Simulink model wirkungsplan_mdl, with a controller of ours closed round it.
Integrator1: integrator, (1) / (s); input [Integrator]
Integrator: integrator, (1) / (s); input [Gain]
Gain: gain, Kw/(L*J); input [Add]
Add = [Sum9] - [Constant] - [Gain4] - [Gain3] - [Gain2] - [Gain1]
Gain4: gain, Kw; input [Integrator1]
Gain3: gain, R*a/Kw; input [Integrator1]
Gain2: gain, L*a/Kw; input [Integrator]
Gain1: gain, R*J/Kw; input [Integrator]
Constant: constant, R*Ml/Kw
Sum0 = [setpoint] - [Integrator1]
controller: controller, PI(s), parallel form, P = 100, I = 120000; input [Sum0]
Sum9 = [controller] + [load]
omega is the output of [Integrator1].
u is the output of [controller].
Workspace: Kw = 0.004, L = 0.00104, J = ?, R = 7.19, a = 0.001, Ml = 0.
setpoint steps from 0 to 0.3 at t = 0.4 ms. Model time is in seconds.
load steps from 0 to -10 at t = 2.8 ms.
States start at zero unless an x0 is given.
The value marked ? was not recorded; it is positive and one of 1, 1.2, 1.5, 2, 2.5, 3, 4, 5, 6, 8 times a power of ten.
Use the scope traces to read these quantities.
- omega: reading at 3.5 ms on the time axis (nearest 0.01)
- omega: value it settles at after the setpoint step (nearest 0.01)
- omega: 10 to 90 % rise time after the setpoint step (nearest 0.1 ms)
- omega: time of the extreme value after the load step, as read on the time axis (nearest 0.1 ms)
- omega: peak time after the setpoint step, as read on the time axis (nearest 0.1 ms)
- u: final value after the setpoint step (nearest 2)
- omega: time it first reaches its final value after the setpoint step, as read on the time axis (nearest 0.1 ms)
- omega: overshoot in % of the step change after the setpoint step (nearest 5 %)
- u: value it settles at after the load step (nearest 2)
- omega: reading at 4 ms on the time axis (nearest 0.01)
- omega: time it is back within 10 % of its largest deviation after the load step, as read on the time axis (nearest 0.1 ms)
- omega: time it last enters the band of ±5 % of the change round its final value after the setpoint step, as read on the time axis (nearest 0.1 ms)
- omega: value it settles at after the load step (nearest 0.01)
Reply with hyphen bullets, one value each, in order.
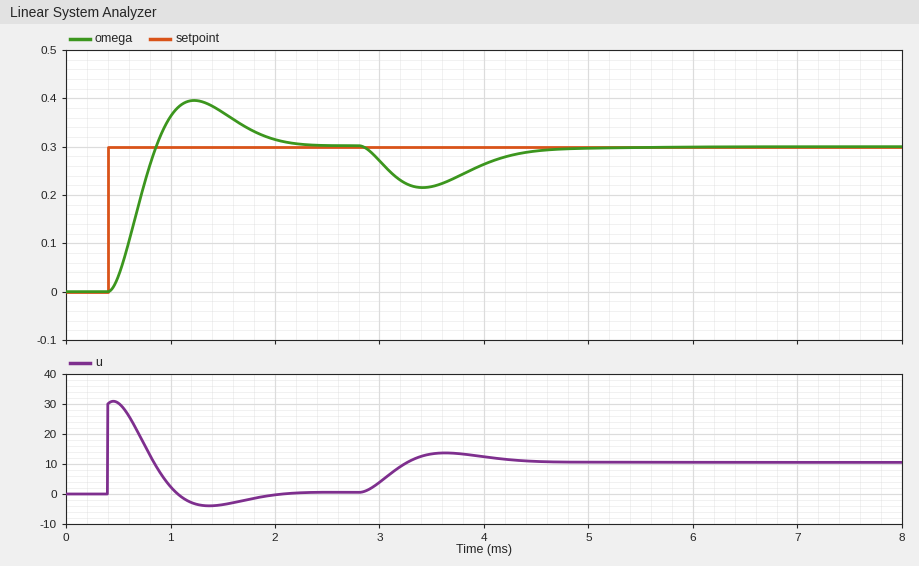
- 0.22
- 0.30
- 0.3 ms
- 3.4 ms
- 1.2 ms
- 0
- 0.9 ms
- 30 %
- 10
- 0.26
- 4.5 ms
- 2.0 ms
- 0.30
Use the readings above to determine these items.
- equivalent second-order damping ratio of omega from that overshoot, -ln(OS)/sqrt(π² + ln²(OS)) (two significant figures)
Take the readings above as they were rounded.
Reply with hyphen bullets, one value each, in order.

- 0.36
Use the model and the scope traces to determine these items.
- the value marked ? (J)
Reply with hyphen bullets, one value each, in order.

- 1.5e-05
